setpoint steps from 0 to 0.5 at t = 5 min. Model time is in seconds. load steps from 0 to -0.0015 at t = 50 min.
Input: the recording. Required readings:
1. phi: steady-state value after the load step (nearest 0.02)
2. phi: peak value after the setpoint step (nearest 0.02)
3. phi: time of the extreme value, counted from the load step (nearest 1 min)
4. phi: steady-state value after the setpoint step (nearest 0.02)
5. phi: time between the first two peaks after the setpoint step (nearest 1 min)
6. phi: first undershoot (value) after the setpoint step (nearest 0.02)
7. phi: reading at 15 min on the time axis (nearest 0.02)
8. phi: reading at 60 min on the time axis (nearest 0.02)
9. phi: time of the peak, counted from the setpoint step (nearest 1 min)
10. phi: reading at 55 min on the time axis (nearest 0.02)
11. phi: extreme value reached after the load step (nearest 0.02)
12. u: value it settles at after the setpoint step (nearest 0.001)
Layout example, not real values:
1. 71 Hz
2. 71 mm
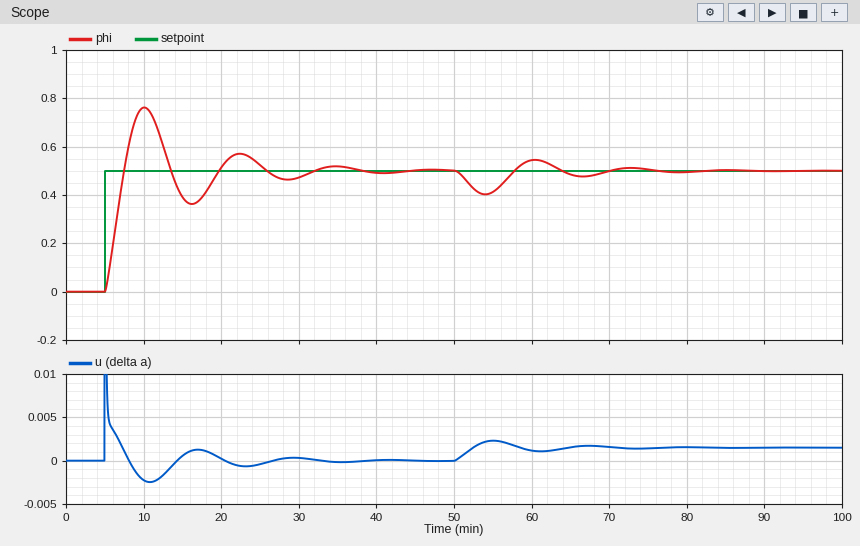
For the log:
1. 0.50
2. 0.76
3. 4 min
4. 0.50
5. 12 min
6. 0.36
7. 0.40
8. 0.54
9. 5 min
10. 0.42
11. 0.40
12. 0.000
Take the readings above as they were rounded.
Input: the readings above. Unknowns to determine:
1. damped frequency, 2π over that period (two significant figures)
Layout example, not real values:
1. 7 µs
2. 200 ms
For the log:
1. 0.52 rad/min
